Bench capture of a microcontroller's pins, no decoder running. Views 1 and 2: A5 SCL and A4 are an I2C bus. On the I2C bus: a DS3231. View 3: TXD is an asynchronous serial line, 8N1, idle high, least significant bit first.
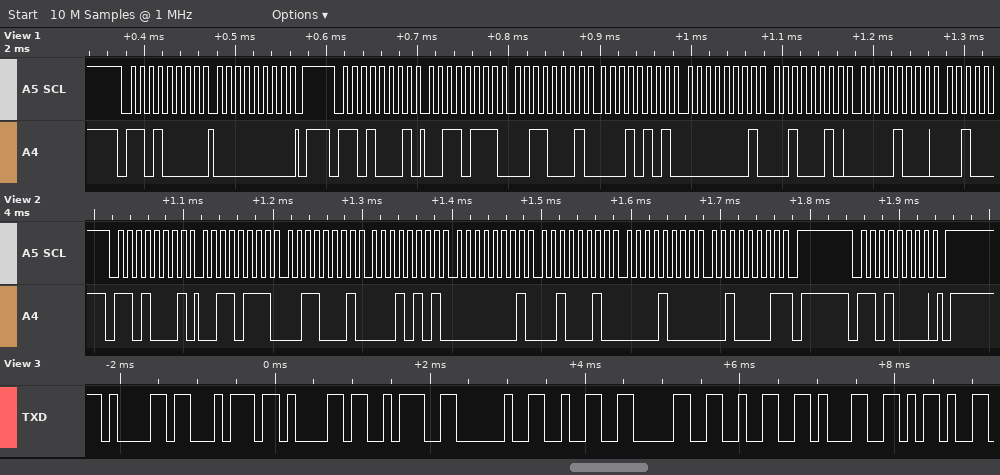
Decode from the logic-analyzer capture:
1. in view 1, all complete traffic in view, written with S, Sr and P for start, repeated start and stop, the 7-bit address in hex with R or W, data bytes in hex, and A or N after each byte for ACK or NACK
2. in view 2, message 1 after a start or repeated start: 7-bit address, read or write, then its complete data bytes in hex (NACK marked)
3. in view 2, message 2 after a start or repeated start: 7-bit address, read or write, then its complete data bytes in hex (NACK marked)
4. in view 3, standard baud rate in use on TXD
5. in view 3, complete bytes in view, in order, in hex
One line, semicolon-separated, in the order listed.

S 68W A 00 A P S 68R A 37 A 31 A 15 A 01 A 22 A 08 A; 0x68 read: 37 31 15 01 22 08 21 NACK; 0x68 write; 9600 baud; 61 74 61 3A 20 32 30 32 31 2D
